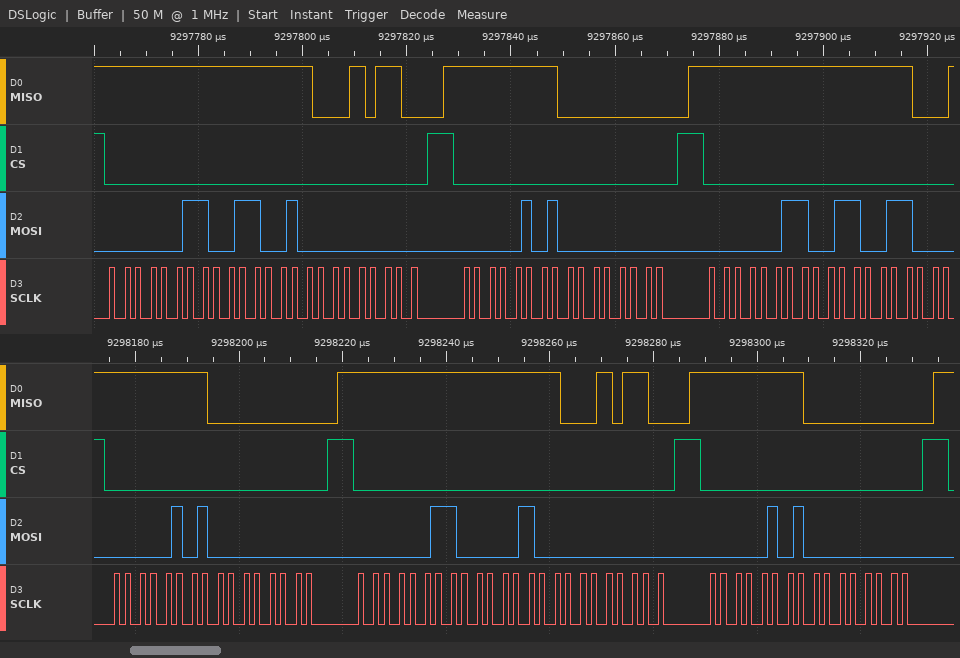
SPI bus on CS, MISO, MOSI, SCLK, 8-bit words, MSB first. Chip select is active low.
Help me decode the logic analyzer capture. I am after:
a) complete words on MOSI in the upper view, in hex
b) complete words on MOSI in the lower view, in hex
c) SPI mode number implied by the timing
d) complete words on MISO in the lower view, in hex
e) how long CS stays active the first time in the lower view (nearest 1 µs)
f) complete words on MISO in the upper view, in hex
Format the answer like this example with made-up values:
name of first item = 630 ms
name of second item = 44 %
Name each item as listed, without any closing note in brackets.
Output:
complete words on MOSI in the upper view, in hex = 03, 32, 00, 05, 00, 03, 33
complete words on MOSI in the lower view, in hex = 05, 00, 03, 04, 00, 05, 00
SPI mode number implied by the timing = 0
complete words on MISO in the lower view, in hex = FF, 00, FF, FF, 16, FF, 00
how long CS stays active the first time in the lower view = 43 µs
complete words on MISO in the upper view, in hex = FF, FF, 16, FF, 00, FF, FF
